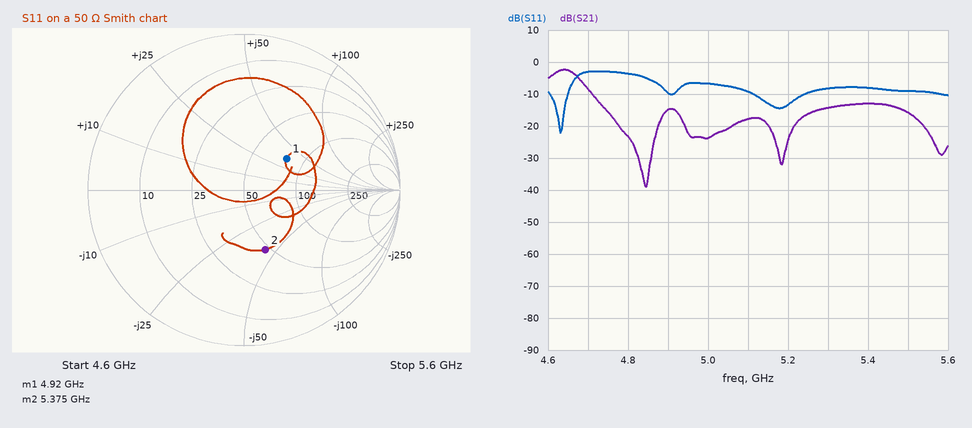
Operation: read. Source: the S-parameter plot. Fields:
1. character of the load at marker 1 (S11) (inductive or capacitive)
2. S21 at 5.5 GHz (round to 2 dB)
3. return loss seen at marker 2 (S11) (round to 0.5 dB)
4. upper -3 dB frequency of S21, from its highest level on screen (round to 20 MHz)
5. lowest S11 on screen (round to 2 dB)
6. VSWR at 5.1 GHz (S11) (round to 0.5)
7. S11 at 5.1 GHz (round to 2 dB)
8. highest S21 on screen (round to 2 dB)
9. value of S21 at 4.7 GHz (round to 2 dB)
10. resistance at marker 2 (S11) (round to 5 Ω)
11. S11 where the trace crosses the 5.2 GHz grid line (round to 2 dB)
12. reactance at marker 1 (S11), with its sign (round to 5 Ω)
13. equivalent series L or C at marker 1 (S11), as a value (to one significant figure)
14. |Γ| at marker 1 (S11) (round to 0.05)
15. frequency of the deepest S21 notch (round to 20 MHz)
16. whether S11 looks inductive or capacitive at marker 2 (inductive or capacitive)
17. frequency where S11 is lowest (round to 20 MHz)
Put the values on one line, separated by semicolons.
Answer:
inductive; -16 dB; 8.0 dB; 4.68 GHz; -22 dB; 2.0; -10 dB; -2 dB; -8 dB; 45 Ω; -14 dB; +35 Ω; 1 nH; 0.35; 4.84 GHz; capacitive; 4.64 GHz
